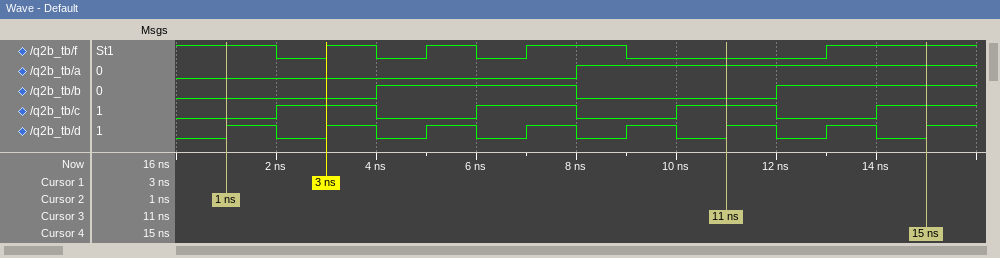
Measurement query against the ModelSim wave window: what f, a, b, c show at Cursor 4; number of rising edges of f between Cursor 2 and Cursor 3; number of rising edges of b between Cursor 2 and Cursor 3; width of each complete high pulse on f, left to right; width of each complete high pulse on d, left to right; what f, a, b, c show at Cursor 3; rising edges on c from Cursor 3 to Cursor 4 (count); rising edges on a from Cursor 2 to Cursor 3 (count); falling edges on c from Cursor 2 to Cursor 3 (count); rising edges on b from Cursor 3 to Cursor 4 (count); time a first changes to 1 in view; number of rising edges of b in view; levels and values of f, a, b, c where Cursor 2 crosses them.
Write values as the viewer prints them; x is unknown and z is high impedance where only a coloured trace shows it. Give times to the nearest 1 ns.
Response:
f=1, a=1, b=1, c=1
3
1
1 ns, 1 ns, 2 ns
1 ns, 1 ns, 1 ns, 1 ns, 1 ns, 1 ns, 1 ns
f=0, a=1, b=0, c=1
1
1
2
1
8 ns
2
f=1, a=0, b=0, c=0
